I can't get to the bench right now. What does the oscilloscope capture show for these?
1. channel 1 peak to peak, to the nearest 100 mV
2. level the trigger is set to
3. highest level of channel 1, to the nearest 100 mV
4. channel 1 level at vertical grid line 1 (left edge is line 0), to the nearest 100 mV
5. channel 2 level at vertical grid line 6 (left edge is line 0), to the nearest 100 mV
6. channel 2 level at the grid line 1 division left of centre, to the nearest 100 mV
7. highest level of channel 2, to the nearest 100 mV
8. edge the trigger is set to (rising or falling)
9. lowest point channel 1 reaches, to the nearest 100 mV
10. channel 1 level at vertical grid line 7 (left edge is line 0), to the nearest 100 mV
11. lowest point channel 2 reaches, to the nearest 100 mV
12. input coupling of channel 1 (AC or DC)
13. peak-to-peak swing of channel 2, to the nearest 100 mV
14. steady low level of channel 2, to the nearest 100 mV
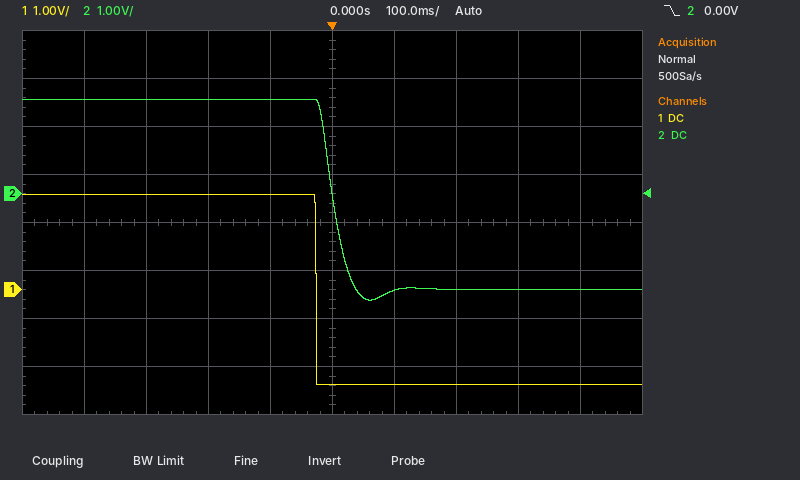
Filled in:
4.0 V
0.00 V
2.0 V
2.0 V
-2.0 V
2.0 V
2.0 V
falling
-2.0 V
-2.0 V
-2.2 V
DC
4.2 V
-2.0 V
